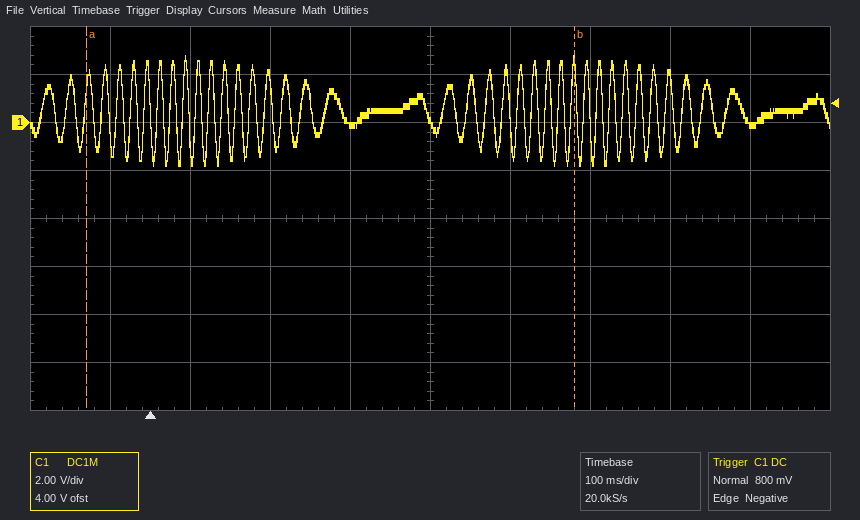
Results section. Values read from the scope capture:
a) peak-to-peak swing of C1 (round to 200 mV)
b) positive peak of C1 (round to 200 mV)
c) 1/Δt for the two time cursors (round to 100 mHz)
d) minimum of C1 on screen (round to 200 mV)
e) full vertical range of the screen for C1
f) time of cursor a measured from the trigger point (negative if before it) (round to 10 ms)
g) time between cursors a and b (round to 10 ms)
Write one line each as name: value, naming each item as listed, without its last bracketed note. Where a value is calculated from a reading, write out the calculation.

peak-to-peak swing of C1: 2.8 V − (-1.8 V) = 4.6 V
positive peak of C1: 2.8 V
1/Δt for the two time cursors: 1 / 610 ms ≈ 1.6 Hz
minimum of C1 on screen: -1.8 V
full vertical range of the screen for C1: 16 V
time of cursor a measured from the trigger point (negative if before it): -80 ms
time between cursors a and b: 610 ms
